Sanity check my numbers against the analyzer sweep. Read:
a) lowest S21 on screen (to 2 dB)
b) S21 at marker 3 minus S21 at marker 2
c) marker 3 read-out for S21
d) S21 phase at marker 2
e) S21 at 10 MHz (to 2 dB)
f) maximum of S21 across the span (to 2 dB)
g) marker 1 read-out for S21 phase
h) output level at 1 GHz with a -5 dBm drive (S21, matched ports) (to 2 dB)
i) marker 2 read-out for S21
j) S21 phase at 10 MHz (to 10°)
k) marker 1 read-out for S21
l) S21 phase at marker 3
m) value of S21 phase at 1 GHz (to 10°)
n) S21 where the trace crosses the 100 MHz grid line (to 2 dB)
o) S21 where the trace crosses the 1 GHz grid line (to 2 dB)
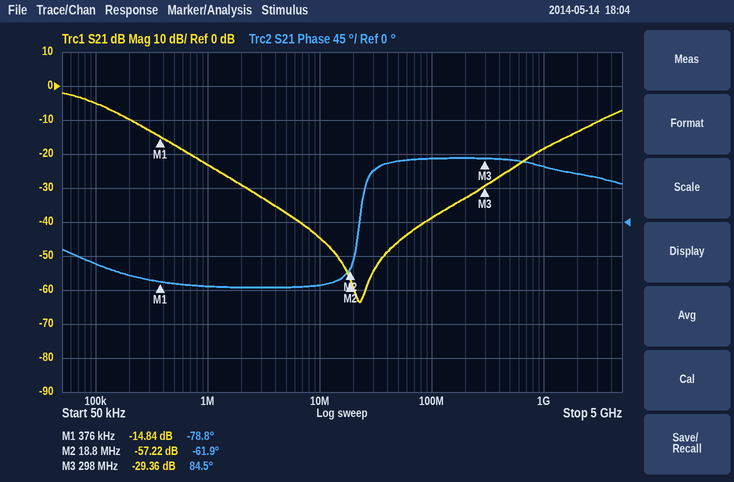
-64 dB
27.86 dB
-29.36 dB
-61.9°
-44 dB
-2 dB
-78.8°
-24 dBm
-57.22 dB
-80°
-14.84 dB
84.5°
70°
-38 dB
-18 dB
